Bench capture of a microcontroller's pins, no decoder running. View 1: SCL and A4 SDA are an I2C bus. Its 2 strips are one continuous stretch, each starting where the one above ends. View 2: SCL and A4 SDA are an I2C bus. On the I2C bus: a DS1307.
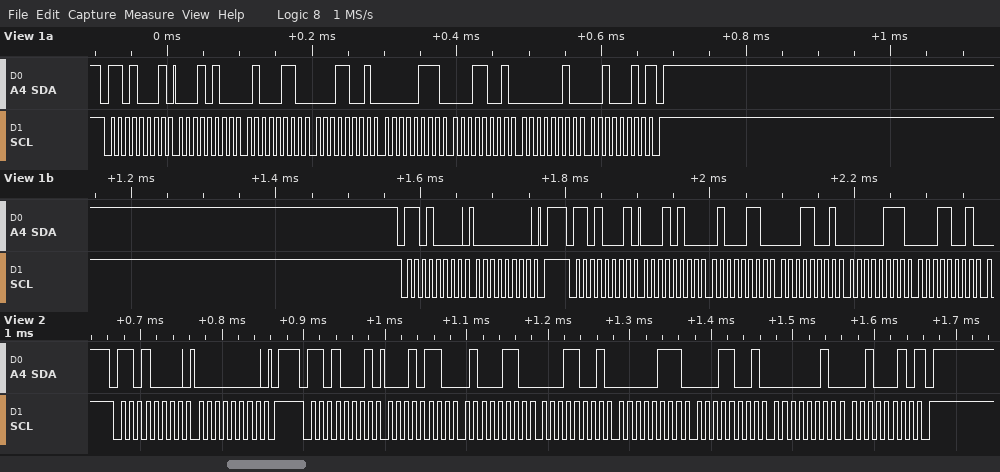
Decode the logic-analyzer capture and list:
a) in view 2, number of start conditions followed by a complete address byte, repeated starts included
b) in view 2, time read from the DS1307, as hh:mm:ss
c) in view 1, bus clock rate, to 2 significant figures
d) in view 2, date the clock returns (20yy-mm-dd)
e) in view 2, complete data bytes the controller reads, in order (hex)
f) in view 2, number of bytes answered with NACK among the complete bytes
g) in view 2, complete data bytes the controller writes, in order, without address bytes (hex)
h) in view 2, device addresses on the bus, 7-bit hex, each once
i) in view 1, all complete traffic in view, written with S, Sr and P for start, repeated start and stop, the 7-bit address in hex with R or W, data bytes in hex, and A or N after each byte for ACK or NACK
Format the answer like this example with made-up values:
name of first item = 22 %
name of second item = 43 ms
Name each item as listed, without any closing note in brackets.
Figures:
in view 2, number of start conditions followed by a complete address byte, repeated starts included = 2
in view 2, time read from the DS1307, as hh:mm:ss = 19:46:16
in view 1, bus clock rate, to 2 significant figures = 100 kHz
in view 2, date the clock returns = 2022-02-19
in view 2, complete data bytes the controller reads, in order = 16 46 19 07 19 02 22
in view 2, number of bytes answered with NACK among the complete bytes = 1
in view 2, complete data bytes the controller writes, in order, without address bytes = 00
in view 2, device addresses on the bus, 7-bit hex, each once = 0x68
in view 1, all complete traffic in view, written with S, Sr and P for start, repeated start and stop, the 7-bit address in hex with R or W, data bytes in hex, and A or N after each byte for ACK or NACK = S 68R A 14 A 46 A 19 A 07 A 19 A 02 A 22 N P S 68W A 00 A P S 68R A 14 A 46 A 19 A 07 A 19 A
